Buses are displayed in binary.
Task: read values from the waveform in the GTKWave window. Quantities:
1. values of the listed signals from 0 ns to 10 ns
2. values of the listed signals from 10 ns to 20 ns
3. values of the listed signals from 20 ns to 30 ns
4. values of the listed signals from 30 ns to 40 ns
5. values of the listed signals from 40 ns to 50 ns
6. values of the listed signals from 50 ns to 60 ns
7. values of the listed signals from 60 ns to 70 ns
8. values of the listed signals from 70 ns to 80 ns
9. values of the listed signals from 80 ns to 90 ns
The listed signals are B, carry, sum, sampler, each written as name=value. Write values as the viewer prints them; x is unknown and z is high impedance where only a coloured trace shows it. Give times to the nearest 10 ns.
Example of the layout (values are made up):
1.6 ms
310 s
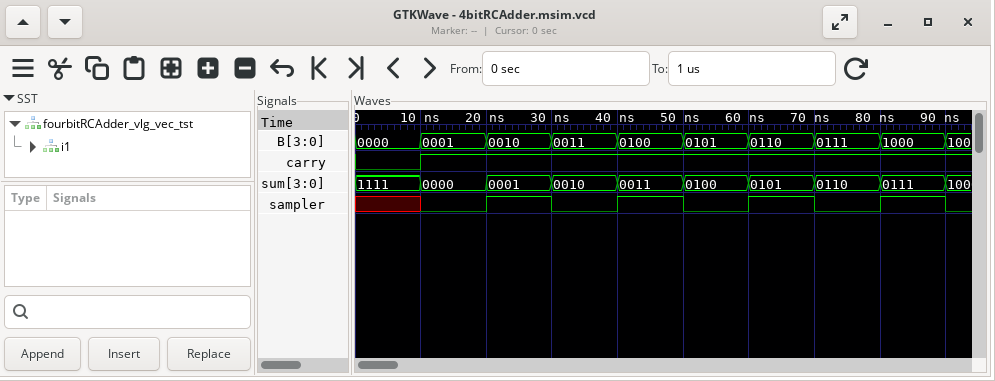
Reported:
B=0000, carry=0, sum=1111, sampler=x
B=0001, carry=1, sum=0000, sampler=0
B=0010, carry=1, sum=0001, sampler=1
B=0011, carry=1, sum=0010, sampler=0
B=0100, carry=1, sum=0011, sampler=1
B=0101, carry=1, sum=0100, sampler=0
B=0110, carry=1, sum=0101, sampler=1
B=0111, carry=1, sum=0110, sampler=0
B=1000, carry=1, sum=0111, sampler=1
